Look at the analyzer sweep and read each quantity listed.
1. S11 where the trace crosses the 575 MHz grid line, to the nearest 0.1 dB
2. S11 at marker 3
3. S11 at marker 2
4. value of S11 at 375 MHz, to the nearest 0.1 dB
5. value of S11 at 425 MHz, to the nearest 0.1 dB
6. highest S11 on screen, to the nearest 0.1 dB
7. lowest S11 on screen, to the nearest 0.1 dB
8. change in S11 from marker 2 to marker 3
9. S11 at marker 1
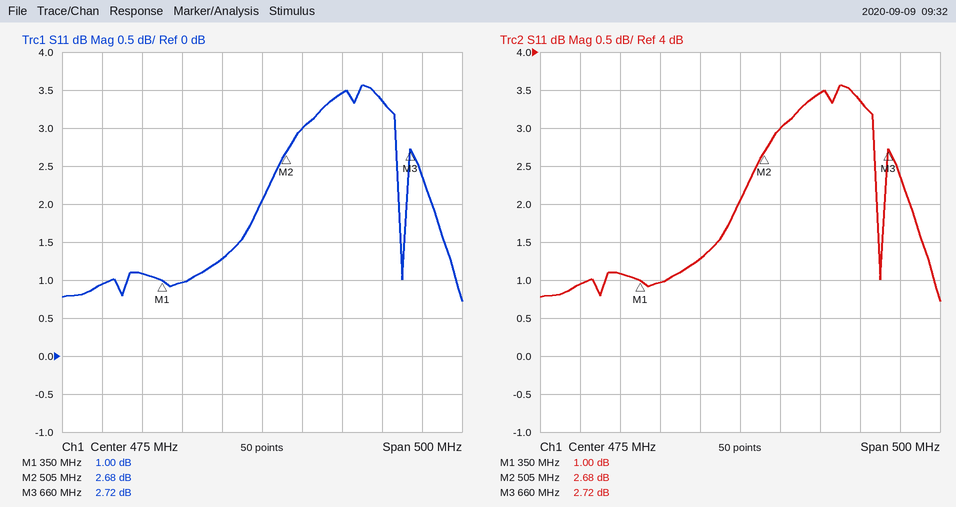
3.5 dB
2.72 dB
2.68 dB
1.0 dB
1.3 dB
3.6 dB
0.7 dB
0.04 dB
1.00 dB
